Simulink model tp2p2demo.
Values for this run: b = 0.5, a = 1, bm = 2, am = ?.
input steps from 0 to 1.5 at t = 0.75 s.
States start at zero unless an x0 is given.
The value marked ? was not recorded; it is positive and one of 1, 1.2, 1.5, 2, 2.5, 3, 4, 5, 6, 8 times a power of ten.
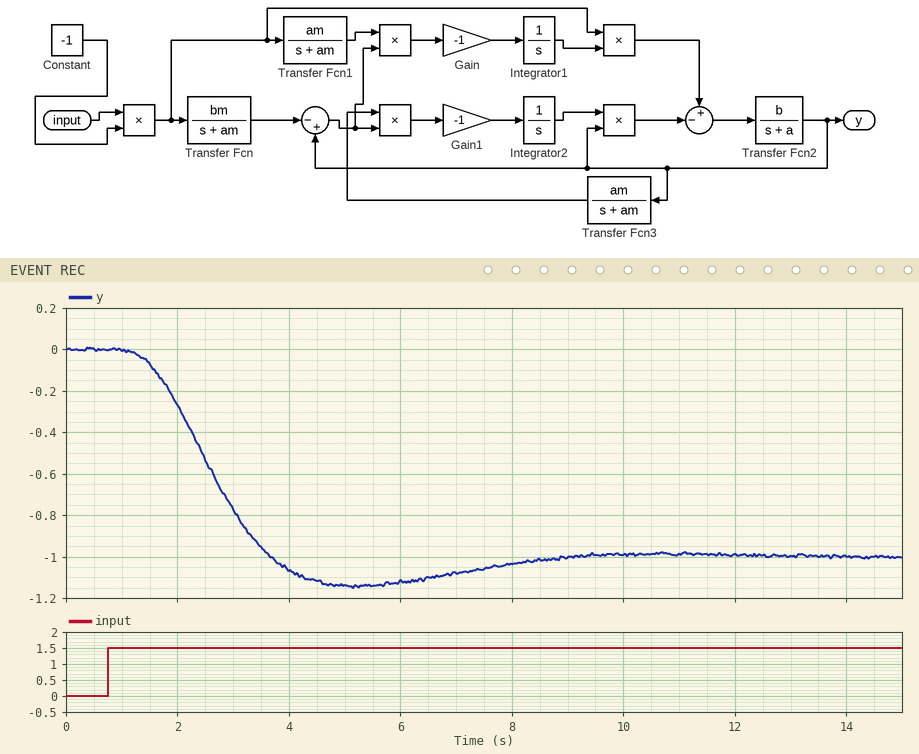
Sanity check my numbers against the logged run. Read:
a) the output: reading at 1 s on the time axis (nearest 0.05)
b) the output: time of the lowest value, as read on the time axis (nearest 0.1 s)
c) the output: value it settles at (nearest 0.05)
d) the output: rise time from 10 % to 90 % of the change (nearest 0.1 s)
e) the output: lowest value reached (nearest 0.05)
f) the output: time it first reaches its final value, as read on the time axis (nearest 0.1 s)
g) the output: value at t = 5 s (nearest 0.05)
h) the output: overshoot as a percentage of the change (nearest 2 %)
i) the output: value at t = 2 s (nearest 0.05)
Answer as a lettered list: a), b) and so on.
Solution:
a) 0.00
b) 5.2 s
c) -1.00
d) 1.7 s
e) -1.15
f) 3.7 s
g) -1.15
h) 14 %
i) -0.25
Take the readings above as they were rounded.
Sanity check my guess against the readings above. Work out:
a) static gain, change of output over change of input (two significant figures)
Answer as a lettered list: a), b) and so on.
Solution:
a) -0.67
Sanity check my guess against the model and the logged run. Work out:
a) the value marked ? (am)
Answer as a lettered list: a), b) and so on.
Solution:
a) 3
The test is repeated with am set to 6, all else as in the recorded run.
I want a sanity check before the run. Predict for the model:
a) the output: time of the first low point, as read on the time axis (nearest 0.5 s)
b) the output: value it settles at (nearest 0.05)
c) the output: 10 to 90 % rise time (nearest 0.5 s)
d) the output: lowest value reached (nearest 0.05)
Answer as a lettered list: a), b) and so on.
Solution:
a) 4.5 s
b) -0.50
c) 1.5 s
d) -0.60
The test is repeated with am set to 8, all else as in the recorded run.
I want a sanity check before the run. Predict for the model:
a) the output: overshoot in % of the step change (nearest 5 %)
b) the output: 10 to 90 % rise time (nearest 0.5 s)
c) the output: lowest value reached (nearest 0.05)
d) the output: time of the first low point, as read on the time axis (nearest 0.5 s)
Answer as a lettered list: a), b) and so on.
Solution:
a) 20 %
b) 1.5 s
c) -0.45
d) 4.5 s
